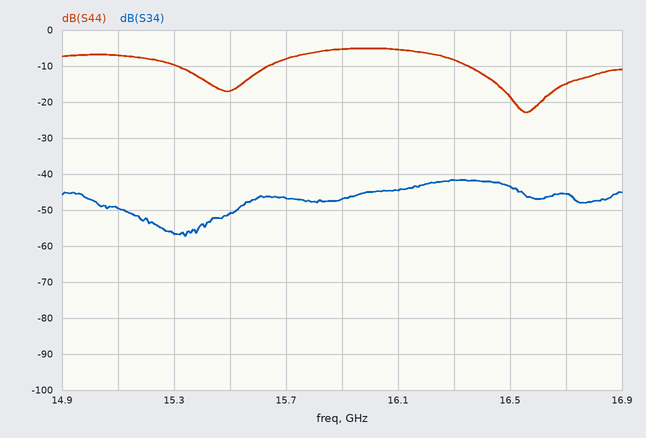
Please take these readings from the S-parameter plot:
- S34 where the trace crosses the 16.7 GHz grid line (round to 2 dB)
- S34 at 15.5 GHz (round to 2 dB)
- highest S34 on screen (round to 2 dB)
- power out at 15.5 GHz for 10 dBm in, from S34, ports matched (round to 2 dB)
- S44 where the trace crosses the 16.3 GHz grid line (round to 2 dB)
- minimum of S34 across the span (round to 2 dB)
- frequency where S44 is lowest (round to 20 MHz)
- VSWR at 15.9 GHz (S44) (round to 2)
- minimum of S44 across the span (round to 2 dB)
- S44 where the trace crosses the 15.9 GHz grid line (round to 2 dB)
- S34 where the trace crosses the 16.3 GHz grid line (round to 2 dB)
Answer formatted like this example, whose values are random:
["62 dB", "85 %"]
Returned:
["-46 dB", "-50 dB", "-42 dB", "-40 dBm", "-8 dB", "-58 dB", "16.56 GHz", "4", "-22 dB", "-6 dB", "-42 dB"]
